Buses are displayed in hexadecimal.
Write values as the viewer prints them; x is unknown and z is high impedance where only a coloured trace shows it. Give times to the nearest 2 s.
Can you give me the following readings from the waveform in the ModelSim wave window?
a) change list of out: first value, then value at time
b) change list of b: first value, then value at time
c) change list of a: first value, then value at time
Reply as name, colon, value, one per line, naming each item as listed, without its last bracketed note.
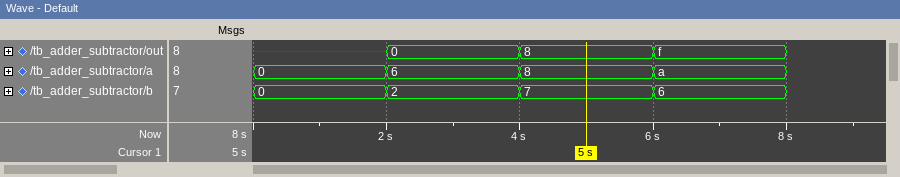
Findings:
change list of out: first value, then value at time: x, 0 at 2 s, 8 at 4 s, f at 6 s
change list of b: first value, then value at time: 0, 2 at 2 s, 7 at 4 s, 6 at 6 s
change list of a: first value, then value at time: 0, 6 at 2 s, 8 at 4 s, a at 6 s
